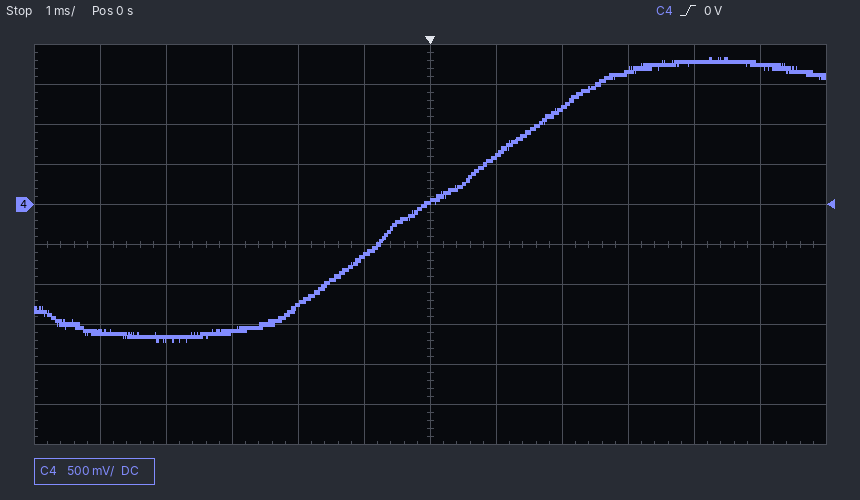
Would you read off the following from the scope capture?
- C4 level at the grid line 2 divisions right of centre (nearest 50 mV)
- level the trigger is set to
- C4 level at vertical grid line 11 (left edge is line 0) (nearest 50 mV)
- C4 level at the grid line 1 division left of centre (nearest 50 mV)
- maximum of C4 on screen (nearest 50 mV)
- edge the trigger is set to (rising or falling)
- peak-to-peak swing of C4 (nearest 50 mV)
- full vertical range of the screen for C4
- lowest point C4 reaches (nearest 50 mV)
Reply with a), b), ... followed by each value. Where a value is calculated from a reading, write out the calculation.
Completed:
a) 1.20 V
b) 0 V
c) 1.75 V
d) -650 mV
e) 1.85 V
f) rising
g) 1.85 V − (-1.70 V) = 3.55 V
h) 5 V
i) -1.70 V
